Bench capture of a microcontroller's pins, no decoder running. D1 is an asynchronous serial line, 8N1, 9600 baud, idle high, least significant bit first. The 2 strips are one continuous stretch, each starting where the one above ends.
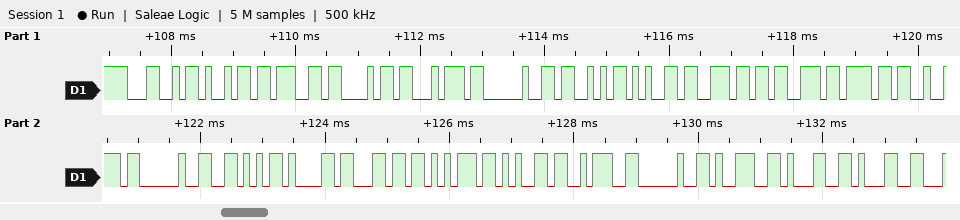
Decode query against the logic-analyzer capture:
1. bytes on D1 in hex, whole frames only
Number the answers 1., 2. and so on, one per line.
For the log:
1. 0x4C 0x69 0x67 0x68 0x74 0x20 0x53 0x65 0x6E 0x73 0x6F 0x72 0x20 0x56 0x61 0x6C 0x75 0x65 0x3A 0x20 0x39 0x31 0x31
